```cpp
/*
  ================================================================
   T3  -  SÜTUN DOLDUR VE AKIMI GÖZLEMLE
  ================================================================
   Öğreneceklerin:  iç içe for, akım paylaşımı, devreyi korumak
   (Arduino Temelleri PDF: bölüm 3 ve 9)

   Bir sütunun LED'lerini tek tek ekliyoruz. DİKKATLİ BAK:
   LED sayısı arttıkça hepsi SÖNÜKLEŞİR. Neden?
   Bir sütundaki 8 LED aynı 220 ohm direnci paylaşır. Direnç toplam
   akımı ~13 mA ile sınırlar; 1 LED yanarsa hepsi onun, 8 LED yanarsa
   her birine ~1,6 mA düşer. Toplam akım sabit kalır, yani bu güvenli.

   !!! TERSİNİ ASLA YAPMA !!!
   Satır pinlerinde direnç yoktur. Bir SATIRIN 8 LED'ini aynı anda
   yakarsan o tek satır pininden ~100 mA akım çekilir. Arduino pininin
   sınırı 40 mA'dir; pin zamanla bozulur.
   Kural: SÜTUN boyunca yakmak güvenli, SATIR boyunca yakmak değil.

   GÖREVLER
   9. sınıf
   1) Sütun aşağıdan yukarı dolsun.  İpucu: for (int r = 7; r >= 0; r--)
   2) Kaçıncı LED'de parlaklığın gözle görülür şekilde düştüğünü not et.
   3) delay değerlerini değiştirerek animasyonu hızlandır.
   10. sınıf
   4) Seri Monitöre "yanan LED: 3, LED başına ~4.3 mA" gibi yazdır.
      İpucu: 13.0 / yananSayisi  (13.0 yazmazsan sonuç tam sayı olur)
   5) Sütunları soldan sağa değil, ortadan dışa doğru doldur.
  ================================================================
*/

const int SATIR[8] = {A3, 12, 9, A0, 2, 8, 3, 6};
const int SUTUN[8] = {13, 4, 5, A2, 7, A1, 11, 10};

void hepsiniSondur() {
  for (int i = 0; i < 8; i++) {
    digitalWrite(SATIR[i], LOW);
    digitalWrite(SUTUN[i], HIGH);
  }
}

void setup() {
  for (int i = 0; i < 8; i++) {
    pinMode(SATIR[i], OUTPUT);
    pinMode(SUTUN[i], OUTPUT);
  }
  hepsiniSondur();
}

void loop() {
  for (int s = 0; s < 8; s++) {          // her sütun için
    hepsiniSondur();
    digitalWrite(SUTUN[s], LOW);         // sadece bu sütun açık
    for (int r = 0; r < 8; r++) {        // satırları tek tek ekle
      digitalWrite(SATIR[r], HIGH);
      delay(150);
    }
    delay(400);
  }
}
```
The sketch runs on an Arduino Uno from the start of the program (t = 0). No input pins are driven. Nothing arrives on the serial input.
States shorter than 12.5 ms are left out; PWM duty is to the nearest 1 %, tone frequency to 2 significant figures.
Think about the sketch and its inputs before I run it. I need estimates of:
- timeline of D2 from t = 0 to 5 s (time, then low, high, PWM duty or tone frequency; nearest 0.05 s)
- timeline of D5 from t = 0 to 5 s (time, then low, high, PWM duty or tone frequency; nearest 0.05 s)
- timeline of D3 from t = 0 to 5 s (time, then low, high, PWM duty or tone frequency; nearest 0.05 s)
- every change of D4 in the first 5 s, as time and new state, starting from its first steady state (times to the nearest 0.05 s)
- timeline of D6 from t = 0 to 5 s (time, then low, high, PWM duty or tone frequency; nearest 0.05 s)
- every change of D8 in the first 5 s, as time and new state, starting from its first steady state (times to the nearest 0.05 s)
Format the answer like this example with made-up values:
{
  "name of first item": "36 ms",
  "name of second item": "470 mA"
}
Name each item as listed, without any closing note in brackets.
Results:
{
  "timeline of D2 from t = 0 to 5 s": "0 s low; 0.6 s high; 1.6 s low; 2.2 s high; 3.2 s low; 3.8 s high; 4.8 s low",
  "timeline of D5 from t = 0 to 5 s": "0 s high; 3.2 s low; 4.8 s high",
  "timeline of D3 from t = 0 to 5 s": "0 s low; 0.9 s high; 1.6 s low; 2.5 s high; 3.2 s low; 4.1 s high; 4.8 s low",
  "every change of D4 in the first 5 s, as time and new state, starting from its first steady state": "0 s high; 1.6 s low; 3.2 s high",
  "timeline of D6 from t = 0 to 5 s": "0 s low; 1.05 s high; 1.6 s low; 2.65 s high; 3.2 s low; 4.25 s high; 4.8 s low",
  "every change of D8 in the first 5 s, as time and new state, starting from its first steady state": "0 s low; 0.75 s high; 1.6 s low; 2.35 s high; 3.2 s low; 3.95 s high; 4.8 s low"
}
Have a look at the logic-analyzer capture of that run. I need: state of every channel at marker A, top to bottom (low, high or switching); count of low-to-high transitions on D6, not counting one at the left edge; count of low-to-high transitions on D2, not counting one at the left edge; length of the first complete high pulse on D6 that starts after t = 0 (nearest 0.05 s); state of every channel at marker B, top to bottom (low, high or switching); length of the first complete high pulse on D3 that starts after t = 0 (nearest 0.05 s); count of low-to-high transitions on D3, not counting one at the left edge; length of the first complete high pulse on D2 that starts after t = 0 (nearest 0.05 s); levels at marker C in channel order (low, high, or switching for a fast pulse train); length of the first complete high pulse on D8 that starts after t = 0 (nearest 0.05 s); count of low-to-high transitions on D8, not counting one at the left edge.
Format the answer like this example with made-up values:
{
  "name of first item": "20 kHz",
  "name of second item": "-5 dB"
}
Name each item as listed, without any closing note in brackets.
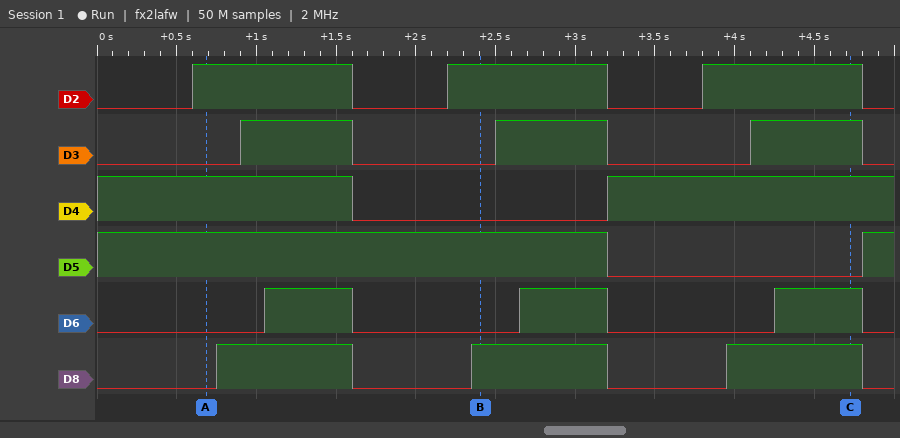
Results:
{
  "state of every channel at marker A, top to bottom": "D2 high, D3 low, D4 high, D5 high, D6 low, D8 low",
  "count of low-to-high transitions on D6, not counting one at the left edge": "3",
  "count of low-to-high transitions on D2, not counting one at the left edge": "3",
  "length of the first complete high pulse on D6 that starts after t = 0": "0.55 s",
  "state of every channel at marker B, top to bottom": "D2 high, D3 low, D4 low, D5 high, D6 low, D8 high",
  "length of the first complete high pulse on D3 that starts after t = 0": "0.70 s",
  "count of low-to-high transitions on D3, not counting one at the left edge": "3",
  "length of the first complete high pulse on D2 that starts after t = 0": "1.00 s",
  "levels at marker C in channel order": "D2 high, D3 high, D4 high, D5 low, D6 high, D8 high",
  "length of the first complete high pulse on D8 that starts after t = 0": "0.85 s",
  "count of low-to-high transitions on D8, not counting one at the left edge": "3"
}
